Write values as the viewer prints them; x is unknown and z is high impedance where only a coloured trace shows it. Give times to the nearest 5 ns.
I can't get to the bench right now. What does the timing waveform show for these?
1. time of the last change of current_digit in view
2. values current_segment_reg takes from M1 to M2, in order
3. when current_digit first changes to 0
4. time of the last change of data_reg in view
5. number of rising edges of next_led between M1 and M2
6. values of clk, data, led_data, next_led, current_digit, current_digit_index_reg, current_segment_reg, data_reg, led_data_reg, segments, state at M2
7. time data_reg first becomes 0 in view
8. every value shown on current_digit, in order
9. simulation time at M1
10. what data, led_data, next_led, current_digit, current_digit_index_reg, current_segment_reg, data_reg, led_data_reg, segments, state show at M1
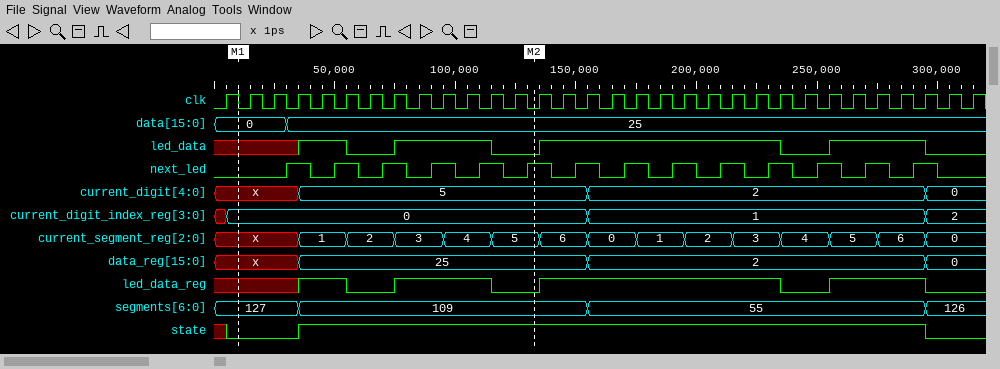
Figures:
295 ns
x, 1, 2, 3, 4, 5
295 ns
295 ns
6
clk=0, data=25, led_data=0, next_led=1, current_digit=5, current_digit_index_reg=0, current_segment_reg=5, data_reg=25, led_data_reg=0, segments=109, state=1
295 ns
x, 5, 2, 0
10 ns
data=0, led_data=x, next_led=0, current_digit=x, current_digit_index_reg=0, current_segment_reg=x, data_reg=x, led_data_reg=x, segments=127, state=0
